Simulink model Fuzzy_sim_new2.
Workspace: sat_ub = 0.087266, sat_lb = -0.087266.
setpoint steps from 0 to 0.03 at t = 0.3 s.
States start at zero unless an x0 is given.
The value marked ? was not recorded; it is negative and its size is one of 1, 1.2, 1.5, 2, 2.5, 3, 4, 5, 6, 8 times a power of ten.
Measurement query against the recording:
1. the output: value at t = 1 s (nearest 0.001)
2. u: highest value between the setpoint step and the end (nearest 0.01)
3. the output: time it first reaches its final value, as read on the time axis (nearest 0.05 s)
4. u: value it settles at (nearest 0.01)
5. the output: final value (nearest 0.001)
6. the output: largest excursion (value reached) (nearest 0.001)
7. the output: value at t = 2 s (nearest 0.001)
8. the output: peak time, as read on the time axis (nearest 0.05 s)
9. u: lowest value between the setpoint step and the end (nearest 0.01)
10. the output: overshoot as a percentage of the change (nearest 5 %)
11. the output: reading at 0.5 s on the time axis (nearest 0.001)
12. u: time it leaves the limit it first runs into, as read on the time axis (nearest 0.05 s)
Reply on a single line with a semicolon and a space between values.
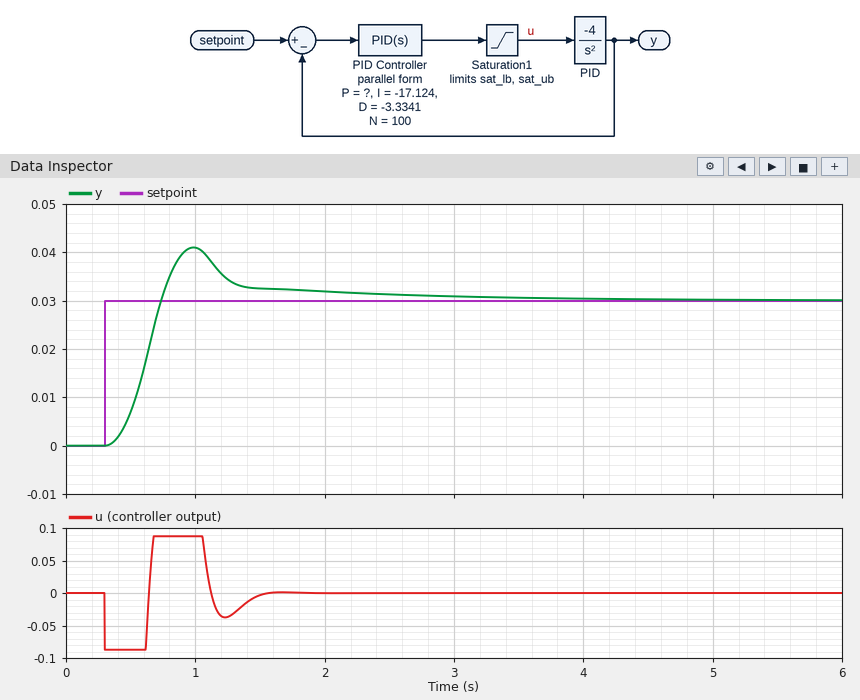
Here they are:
0.041; 0.09; 0.75 s; 0.00; 0.030; 0.041; 0.032; 1.00 s; -0.09; 35 %; 0.007; 0.60 s
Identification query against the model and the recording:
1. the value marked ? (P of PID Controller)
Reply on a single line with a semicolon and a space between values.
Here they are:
-25
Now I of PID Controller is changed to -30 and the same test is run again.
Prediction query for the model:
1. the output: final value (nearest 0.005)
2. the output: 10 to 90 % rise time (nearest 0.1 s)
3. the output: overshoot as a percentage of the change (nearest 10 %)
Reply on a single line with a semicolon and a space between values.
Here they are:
0.030; 0.3 s; 60 %
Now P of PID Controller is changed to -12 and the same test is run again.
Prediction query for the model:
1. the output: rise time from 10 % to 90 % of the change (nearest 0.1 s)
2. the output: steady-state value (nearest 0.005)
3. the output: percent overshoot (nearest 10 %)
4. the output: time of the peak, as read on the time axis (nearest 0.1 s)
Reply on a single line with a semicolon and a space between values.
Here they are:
0.3 s; 0.030; 30 %; 1.2 s
